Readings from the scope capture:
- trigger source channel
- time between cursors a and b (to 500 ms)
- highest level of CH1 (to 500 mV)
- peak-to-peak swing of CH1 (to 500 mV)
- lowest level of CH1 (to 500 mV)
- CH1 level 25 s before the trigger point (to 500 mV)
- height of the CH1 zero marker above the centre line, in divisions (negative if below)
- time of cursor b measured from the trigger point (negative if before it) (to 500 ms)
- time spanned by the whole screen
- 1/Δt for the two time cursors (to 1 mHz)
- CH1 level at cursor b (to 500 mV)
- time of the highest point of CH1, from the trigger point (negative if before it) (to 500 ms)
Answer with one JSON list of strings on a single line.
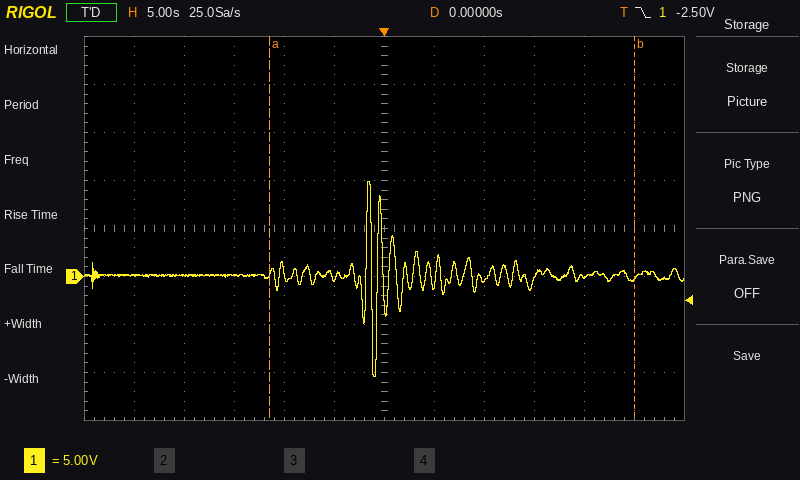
["CH1", "36.5 s", "10.0 V", "20.5 V", "-10.5 V", "0.0 V", "-1.0 div", "+25.0 s", "60 s", "27 mHz", "0.0 V", "-1.5 s"]
